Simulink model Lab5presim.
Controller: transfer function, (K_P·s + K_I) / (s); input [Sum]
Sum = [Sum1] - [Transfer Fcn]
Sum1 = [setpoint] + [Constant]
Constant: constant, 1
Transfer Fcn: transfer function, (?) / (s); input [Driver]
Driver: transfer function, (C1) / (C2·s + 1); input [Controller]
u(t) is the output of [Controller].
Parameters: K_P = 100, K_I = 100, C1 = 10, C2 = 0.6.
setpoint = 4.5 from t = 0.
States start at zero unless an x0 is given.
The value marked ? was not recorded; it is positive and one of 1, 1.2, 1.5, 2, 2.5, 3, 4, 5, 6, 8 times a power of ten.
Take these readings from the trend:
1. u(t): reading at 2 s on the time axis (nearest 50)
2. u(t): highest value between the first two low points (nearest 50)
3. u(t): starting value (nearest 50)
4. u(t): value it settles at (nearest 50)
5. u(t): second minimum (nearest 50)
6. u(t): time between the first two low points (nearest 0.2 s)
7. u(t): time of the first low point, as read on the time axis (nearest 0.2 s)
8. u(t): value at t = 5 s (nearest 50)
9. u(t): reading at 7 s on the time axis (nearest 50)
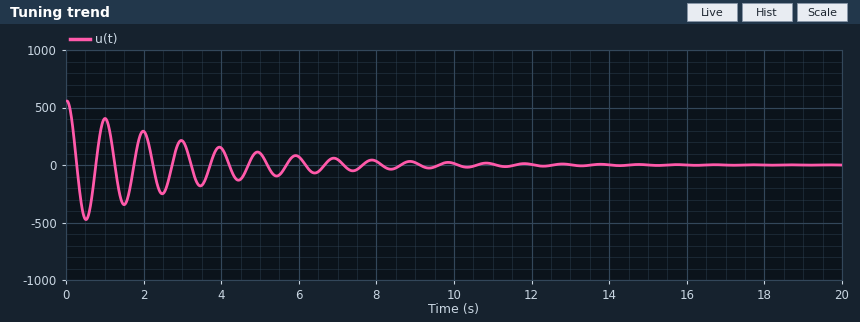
300
400
550
0
-350
1.0 s
0.6 s
100
50
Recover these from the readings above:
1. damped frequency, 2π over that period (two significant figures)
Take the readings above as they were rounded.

6.3 rad/s
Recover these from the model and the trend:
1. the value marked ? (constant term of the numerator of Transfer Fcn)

0.025
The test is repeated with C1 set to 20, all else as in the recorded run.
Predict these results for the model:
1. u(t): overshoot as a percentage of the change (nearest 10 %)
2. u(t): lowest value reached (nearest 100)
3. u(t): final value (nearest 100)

90 %
-500
0
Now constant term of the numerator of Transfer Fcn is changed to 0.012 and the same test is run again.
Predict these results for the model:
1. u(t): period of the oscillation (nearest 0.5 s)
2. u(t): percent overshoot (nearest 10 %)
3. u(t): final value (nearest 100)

1.5 s
80 %
0
